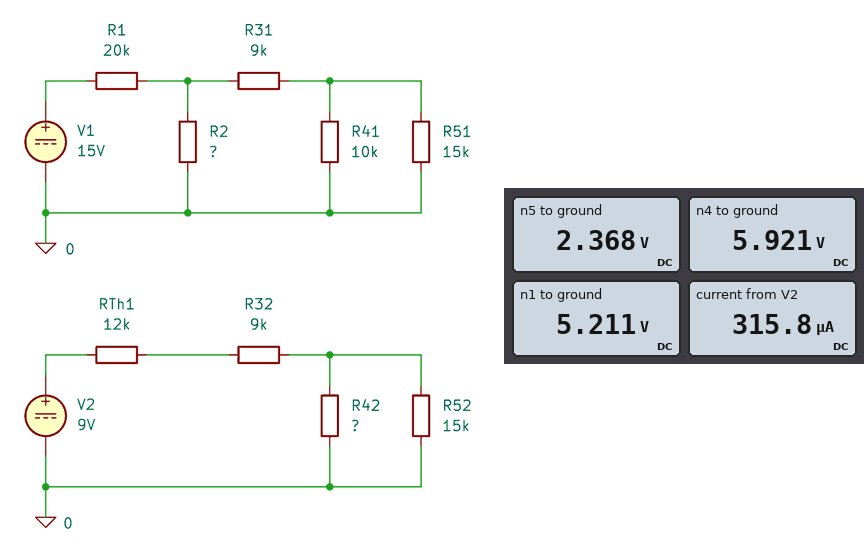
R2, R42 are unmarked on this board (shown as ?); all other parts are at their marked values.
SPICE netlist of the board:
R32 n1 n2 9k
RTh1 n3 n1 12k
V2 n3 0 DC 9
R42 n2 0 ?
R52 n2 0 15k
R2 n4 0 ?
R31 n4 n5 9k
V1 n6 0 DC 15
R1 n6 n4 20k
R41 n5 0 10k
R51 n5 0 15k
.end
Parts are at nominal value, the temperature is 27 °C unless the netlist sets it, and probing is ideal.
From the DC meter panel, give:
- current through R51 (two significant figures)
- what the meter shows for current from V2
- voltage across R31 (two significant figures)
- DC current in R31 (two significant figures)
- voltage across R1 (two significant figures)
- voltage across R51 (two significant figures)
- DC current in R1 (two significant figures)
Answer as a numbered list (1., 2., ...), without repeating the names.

1. 160 µA
2. 315.8 µA
3. 3.6 V
4. 390 µA
5. 9.1 V
6. 2.4 V
7. 450 µA
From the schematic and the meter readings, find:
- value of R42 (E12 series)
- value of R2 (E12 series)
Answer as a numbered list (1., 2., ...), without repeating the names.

1. 15 kΩ
2. 100 kΩ
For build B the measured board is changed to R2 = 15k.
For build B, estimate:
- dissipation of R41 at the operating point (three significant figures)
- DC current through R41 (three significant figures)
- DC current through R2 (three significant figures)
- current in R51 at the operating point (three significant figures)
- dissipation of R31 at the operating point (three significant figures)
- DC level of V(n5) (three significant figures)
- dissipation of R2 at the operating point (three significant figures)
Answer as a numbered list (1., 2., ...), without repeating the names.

1. 268 µW
2. 164 µA
3. 273 µA
4. 109 µA
5. 669 µW
6. 1.64 V
7. 1.12 mW
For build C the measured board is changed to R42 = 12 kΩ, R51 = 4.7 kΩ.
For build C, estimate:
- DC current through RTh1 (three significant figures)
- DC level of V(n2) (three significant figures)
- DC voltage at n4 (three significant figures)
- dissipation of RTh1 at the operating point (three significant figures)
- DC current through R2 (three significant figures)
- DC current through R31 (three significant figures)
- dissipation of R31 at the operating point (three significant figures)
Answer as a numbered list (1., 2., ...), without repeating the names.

1. 325 µA
2. 2.17 V
3. 5.28 V
4. 1.27 mW
5. 52.8 µA
6. 433 µA
7. 1.69 mW
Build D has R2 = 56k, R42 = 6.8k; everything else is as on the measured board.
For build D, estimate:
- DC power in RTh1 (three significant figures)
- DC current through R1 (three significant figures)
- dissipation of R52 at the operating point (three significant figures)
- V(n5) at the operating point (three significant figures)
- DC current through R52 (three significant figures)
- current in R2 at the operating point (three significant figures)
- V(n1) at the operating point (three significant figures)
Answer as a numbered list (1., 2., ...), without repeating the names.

1. 1.47 mW
2. 471 µA
3. 179 µW
4. 2.23 V
5. 109 µA
6. 99.6 µA
7. 4.79 V
